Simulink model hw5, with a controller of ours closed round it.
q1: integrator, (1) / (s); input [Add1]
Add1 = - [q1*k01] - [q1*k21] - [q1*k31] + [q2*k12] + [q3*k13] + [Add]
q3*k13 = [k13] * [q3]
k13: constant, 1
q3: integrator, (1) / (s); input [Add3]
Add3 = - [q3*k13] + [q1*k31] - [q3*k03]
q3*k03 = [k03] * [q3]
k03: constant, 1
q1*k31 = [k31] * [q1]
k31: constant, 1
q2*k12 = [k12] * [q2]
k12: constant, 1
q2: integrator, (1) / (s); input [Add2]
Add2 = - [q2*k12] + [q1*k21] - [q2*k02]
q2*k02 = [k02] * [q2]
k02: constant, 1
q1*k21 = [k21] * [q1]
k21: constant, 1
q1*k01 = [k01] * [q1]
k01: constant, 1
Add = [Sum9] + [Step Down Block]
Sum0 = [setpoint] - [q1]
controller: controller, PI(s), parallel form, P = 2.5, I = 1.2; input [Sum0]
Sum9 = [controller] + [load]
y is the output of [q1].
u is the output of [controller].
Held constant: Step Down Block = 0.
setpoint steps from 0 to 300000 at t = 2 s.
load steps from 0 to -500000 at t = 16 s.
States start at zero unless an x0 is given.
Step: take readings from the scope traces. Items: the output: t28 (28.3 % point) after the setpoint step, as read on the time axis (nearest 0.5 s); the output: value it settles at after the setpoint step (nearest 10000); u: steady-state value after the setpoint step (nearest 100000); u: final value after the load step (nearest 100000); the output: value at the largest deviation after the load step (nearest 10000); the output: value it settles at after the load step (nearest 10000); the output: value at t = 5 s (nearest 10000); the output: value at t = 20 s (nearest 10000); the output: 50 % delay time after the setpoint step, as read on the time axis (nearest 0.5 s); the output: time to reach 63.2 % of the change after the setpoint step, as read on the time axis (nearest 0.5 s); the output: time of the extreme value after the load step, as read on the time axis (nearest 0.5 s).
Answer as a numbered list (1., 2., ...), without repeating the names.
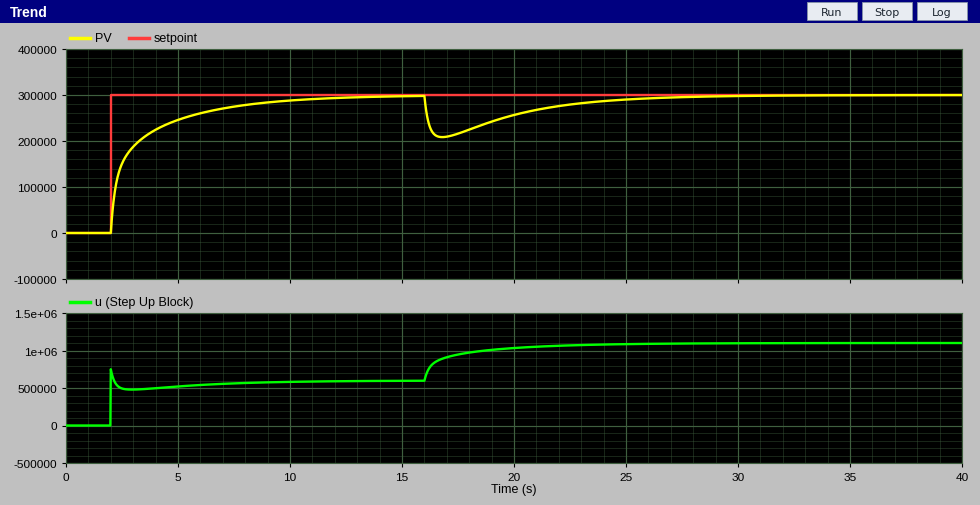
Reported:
1. 2.0 s
2. 300000
3. 600000
4. 1100000
5. 210000
6. 300000
7. 250000
8. 260000
9. 2.5 s
10. 3.0 s
11. 17.0 s
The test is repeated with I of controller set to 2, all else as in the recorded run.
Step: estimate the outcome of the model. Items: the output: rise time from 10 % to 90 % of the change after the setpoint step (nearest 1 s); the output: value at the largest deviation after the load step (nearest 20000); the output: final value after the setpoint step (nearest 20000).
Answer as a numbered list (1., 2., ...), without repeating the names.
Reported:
1. 3 s
2. 220000
3. 300000
